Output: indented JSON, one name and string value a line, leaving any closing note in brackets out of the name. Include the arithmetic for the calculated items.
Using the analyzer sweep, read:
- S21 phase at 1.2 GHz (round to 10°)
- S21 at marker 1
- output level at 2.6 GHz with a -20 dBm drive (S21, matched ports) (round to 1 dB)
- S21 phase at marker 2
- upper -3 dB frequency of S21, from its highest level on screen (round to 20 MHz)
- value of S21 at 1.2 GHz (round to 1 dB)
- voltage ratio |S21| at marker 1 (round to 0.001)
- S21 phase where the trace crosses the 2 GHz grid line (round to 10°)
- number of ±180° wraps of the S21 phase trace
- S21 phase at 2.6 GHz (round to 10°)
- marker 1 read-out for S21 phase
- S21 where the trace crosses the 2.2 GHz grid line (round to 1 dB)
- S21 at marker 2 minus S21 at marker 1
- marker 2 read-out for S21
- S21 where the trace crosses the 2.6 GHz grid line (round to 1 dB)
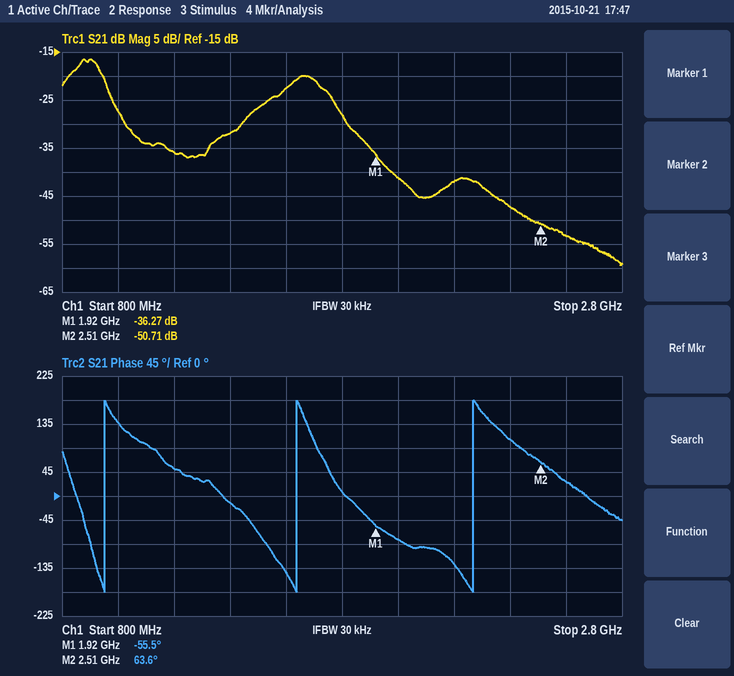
{
  "S21 phase at 1.2 GHz": "50°",
  "S21 at marker 1": "-36.27 dB",
  "output level at 2.6 GHz with a -20 dBm drive (S21, matched ports)": "-20 dBm + (-53 dB) = -73 dBm",
  "S21 phase at marker 2": "63.6°",
  "upper -3 dB frequency of S21, from its highest level on screen": "940 MHz",
  "value of S21 at 1.2 GHz": "-36 dB",
  "voltage ratio |S21| at marker 1": "10^(-36.27/20) ≈ 0.015",
  "S21 phase where the trace crosses the 2 GHz grid line": "-80°",
  "number of ±180° wraps of the S21 phase trace": "3",
  "S21 phase at 2.6 GHz": "30°",
  "marker 1 read-out for S21 phase": "-55.5°",
  "S21 where the trace crosses the 2.2 GHz grid line": "-42 dB",
  "S21 at marker 2 minus S21 at marker 1": "-50.71 − (-36.27) = -14.44 dB",
  "marker 2 read-out for S21": "-50.71 dB",
  "S21 where the trace crosses the 2.6 GHz grid line": "-53 dB"
}
